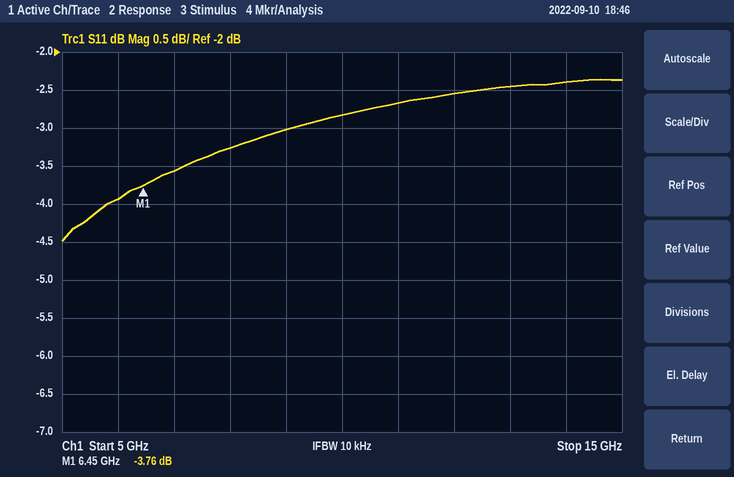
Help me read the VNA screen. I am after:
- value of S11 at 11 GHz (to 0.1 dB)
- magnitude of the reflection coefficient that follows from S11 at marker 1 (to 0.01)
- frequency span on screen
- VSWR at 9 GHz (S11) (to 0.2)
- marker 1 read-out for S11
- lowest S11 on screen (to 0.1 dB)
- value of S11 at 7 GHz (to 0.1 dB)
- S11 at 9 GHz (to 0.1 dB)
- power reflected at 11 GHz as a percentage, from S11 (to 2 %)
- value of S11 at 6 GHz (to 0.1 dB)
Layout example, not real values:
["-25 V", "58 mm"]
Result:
["-2.7 dB", "0.65", "10 GHz", "5.8", "-3.76 dB", "-4.5 dB", "-3.6 dB", "-3.0 dB", "54 %", "-3.9 dB"]
